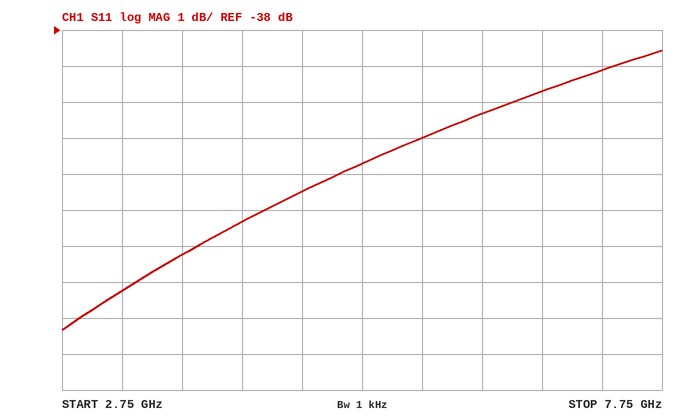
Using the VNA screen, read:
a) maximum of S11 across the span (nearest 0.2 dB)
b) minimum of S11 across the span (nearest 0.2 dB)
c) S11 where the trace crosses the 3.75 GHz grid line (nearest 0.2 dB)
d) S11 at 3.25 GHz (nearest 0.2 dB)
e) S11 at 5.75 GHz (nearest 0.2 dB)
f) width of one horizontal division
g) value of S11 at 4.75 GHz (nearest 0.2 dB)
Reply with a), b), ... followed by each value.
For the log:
a) -38.6 dB
b) -46.4 dB
c) -44.2 dB
d) -45.2 dB
e) -41.0 dB
f) 500 MHz
g) -42.4 dB
